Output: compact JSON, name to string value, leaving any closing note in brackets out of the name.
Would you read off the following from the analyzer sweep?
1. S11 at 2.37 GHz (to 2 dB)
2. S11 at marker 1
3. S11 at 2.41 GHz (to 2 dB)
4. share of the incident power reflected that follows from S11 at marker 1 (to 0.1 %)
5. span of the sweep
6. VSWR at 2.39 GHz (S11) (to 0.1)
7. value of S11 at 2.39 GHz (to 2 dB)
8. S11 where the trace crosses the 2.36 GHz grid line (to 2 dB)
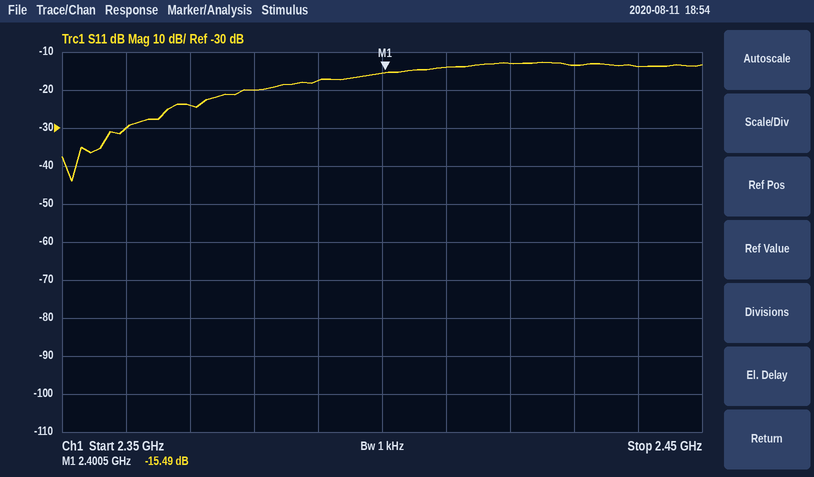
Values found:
{"S11 at 2.37 GHz": "-24 dB", "S11 at marker 1": "-15.49 dB", "S11 at 2.41 GHz": "-14 dB", "share of the incident power reflected that follows from S11 at marker 1": "2.8 %", "span of the sweep": "100 MHz", "VSWR at 2.39 GHz (S11)": "1.3", "value of S11 at 2.39 GHz": "-18 dB", "S11 where the trace crosses the 2.36 GHz grid line": "-30 dB"}
